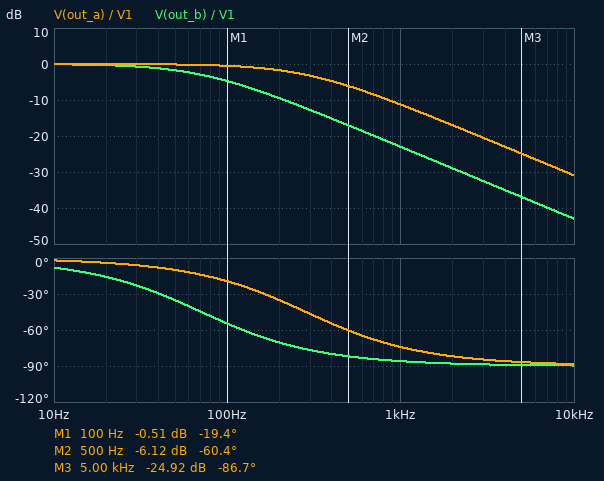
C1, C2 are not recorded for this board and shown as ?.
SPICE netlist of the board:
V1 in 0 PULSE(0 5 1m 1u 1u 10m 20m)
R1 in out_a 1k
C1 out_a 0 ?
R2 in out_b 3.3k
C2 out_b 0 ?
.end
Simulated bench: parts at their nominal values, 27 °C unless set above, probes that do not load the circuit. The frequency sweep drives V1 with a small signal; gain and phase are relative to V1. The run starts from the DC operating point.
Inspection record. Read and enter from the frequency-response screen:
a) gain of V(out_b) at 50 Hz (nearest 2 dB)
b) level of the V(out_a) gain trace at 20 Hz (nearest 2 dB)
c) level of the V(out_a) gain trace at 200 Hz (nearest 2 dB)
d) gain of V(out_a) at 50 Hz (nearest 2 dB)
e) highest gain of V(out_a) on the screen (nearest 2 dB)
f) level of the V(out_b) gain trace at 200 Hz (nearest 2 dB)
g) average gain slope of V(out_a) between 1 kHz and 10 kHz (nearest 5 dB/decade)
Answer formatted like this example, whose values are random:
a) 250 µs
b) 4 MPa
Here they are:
a) -2 dB
b) 0 dB
c) -2 dB
d) 0 dB
e) 0 dB
f) -10 dB
g) -20 dB/decade
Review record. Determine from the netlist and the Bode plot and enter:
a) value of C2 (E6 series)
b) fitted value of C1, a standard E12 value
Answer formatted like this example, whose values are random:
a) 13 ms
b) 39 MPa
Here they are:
a) 680 nF
b) 560 nF
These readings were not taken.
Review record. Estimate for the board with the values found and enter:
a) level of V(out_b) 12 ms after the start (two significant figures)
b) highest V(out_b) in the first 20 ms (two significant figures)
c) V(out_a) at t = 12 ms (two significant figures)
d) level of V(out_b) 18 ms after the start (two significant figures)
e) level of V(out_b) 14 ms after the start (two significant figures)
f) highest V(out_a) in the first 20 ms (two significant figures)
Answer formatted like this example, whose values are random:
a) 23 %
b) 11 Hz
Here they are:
a) 3.2 V
b) 4.9 V
c) 840 mV
d) 220 mV
e) 1.3 V
f) 5.0 V
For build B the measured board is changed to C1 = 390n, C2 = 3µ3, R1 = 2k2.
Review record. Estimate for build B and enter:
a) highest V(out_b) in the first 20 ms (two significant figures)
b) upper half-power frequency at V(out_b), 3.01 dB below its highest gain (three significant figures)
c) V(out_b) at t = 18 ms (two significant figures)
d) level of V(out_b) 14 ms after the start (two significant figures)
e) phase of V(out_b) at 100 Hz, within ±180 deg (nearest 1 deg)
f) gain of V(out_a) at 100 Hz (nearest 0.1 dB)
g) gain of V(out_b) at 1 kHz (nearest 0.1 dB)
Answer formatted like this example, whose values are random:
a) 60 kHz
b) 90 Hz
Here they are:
a) 3.0 V
b) 14.6 Hz
c) 1.6 V
d) 2.3 V
e) -82 deg
f) -1.1 dB
g) -36.7 dB
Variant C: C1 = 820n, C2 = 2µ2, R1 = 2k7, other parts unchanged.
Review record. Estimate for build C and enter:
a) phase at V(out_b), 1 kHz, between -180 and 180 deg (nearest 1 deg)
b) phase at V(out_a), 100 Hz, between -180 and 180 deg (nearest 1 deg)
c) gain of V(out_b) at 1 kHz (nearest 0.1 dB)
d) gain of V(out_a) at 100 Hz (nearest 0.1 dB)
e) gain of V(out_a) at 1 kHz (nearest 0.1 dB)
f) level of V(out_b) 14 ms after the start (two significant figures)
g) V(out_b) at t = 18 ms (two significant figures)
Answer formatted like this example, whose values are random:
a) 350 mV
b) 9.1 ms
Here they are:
a) -89 deg
b) -54 deg
c) -33.2 dB
d) -4.7 dB
e) -22.9 dB
f) 2.5 V
g) 1.4 V
